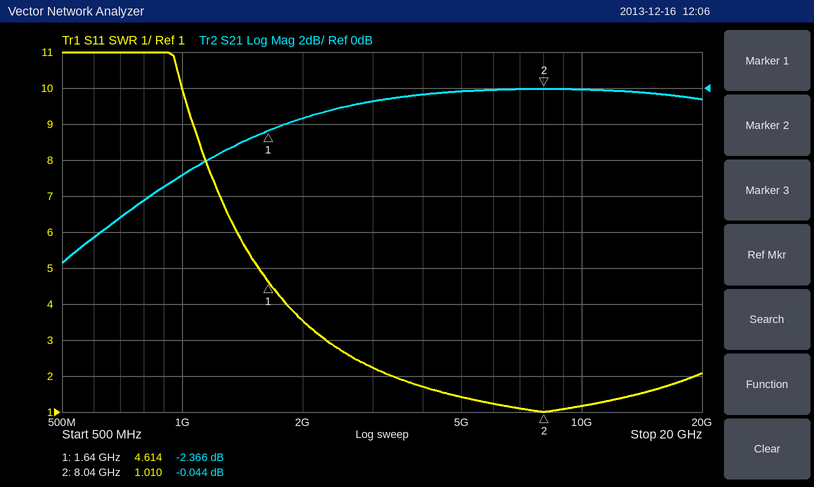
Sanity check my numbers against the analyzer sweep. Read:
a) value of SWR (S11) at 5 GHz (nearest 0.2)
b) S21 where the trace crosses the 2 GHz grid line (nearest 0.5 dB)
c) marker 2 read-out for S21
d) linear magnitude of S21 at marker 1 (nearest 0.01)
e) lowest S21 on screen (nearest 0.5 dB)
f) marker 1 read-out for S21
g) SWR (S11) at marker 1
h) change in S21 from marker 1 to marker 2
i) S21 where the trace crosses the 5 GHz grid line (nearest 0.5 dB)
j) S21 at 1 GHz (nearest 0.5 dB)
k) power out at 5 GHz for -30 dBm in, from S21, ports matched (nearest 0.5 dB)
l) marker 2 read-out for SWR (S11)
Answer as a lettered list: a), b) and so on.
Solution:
a) 1.4
b) -1.5 dB
c) -0.044 dB
d) 0.76
e) -9.5 dB
f) -2.366 dB
g) 4.614
h) 2.322 dB
i) 0.0 dB
j) -5.0 dB
k) -30.0 dBm
l) 1.010
